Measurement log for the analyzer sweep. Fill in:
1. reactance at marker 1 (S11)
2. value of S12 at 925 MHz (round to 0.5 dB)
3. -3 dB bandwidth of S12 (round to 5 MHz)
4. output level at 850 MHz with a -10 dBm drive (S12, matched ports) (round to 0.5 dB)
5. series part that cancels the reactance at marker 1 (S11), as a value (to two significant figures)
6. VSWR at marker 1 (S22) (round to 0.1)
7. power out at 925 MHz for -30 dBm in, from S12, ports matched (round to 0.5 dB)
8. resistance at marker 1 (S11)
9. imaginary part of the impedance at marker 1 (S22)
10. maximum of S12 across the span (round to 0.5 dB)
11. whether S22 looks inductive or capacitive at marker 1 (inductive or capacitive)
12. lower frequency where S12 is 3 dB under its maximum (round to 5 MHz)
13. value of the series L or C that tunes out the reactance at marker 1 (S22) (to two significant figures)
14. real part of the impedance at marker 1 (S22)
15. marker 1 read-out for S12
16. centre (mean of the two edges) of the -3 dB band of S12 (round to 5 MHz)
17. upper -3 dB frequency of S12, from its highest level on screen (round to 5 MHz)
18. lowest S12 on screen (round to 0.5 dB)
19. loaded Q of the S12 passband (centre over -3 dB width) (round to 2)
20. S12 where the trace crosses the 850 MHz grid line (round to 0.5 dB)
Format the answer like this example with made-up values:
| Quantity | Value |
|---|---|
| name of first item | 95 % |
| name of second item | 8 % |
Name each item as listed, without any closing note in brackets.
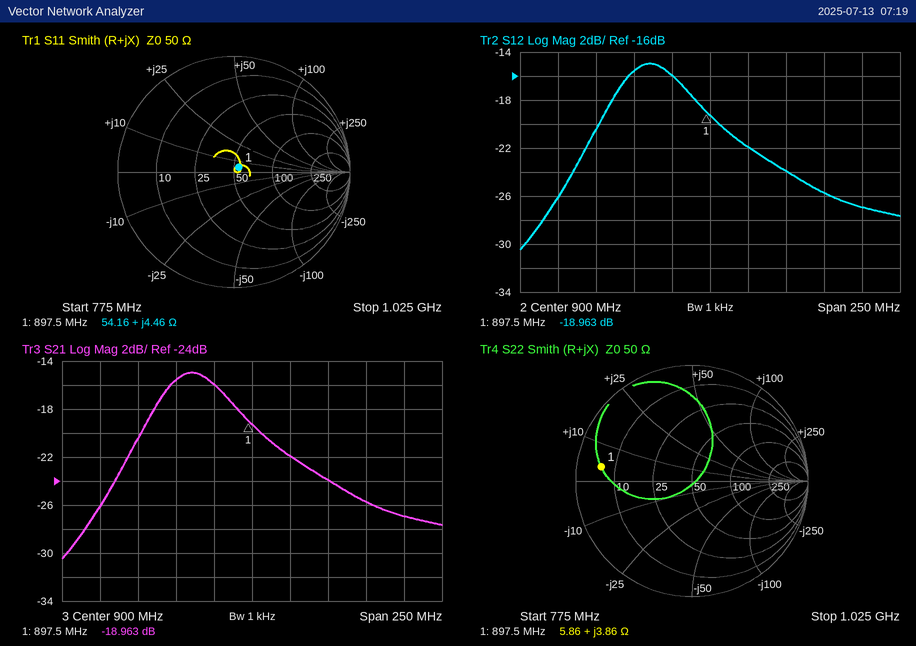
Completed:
| Quantity | Value |
|---|---|
| reactance at marker 1 | +4.46 Ω |
| value of S12 at 925 MHz | -22.0 dB |
| -3 dB bandwidth of S12 | 55 MHz |
| output level at 850 MHz with a -10 dBm drive (S12, matched ports) | -25.5 dBm |
| series part that cancels the reactance at marker 1 (S11), as a value | 40 pF |
| VSWR at marker 1 (S22) | 8.6 |
| power out at 925 MHz for -30 dBm in, from S12, ports matched | -52.0 dBm |
| resistance at marker 1 | 54.16 Ω |
| imaginary part of the impedance at marker 1 | +3.86 Ω |
| maximum of S12 across the span | -15.0 dB |
| whether S22 looks inductive or capacitive at marker 1 | inductive |
| lower frequency where S12 is 3 dB under its maximum | 835 MHz |
| value of the series L or C that tunes out the reactance at marker 1 (S22) | 46 pF |
| real part of the impedance at marker 1 | 5.86 Ω |
| marker 1 read-out for S12 | -18.963 dB |
| centre (mean of the two edges) of the -3 dB band of S12 | 865 MHz |
| upper -3 dB frequency of S12, from its highest level on screen | 890 MHz |
| lowest S12 on screen | -30.5 dB |
| loaded Q of the S12 passband (centre over -3 dB width) | 16 |
| S12 where the trace crosses the 850 MHz grid line | -15.5 dB |
